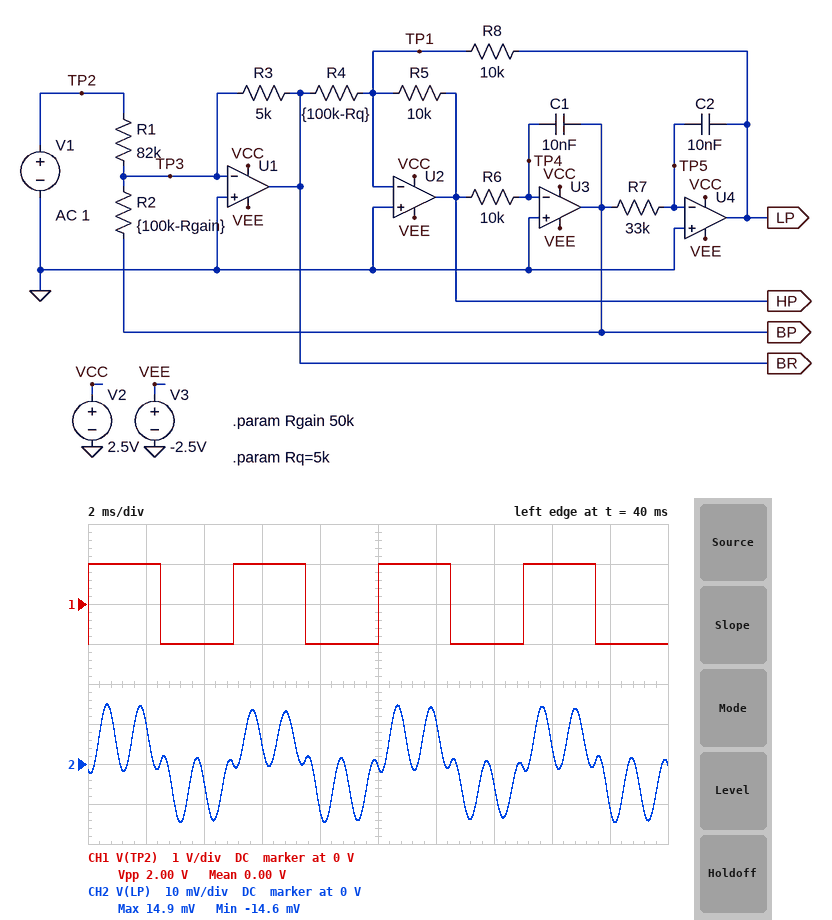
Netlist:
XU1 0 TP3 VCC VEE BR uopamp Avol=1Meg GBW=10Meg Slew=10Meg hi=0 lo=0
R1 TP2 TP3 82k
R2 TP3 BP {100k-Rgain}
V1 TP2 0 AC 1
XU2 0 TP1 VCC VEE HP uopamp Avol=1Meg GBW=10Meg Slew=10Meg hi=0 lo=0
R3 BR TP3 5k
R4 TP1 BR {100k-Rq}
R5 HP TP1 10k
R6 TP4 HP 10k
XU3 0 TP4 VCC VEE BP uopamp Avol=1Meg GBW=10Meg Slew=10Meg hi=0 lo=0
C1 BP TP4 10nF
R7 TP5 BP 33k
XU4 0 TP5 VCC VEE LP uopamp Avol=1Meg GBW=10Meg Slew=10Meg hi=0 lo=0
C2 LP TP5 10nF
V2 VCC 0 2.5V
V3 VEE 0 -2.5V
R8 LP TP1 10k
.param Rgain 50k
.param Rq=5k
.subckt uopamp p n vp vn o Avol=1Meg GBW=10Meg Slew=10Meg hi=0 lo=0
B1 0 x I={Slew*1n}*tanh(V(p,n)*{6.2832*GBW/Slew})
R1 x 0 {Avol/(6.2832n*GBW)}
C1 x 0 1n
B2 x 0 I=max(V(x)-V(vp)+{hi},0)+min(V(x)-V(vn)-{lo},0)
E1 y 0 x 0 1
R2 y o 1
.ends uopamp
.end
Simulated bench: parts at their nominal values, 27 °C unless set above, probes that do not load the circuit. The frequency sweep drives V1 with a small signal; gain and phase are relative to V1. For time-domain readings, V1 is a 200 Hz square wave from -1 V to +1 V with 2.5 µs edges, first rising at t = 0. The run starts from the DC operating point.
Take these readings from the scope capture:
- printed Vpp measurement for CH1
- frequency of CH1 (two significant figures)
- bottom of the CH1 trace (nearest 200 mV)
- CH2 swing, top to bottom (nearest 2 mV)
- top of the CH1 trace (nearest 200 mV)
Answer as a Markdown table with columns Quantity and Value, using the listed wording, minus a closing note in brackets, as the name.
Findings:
| Quantity | Value |
|---|---|
| printed Vpp measurement for CH1 | 2.00 V |
| frequency of CH1 | 200 Hz |
| bottom of the CH1 trace | -1.0 V |
| CH2 swing, top to bottom | 30 mV |
| top of the CH1 trace | 1.0 V |
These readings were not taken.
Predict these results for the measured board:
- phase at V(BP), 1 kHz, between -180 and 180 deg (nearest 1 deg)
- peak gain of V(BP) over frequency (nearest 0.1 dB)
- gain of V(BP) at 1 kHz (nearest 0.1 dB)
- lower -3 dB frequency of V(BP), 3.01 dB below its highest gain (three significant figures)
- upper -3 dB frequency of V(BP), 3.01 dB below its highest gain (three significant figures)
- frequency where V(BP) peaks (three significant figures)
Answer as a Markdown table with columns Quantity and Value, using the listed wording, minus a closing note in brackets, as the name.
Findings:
| Quantity | Value |
|---|---|
| phase at V(BP), 1 kHz, between -180 and 180 deg | 94 deg |
| peak gain of V(BP) over frequency | -4.1 dB |
| gain of V(BP) at 1 kHz | -27.2 dB |
| lower -3 dB frequency of V(BP), 3.01 dB below its highest gain | 868 Hz |
| upper -3 dB frequency of V(BP), 3.01 dB below its highest gain | 884 Hz |
| frequency where V(BP) peaks | 876 Hz |
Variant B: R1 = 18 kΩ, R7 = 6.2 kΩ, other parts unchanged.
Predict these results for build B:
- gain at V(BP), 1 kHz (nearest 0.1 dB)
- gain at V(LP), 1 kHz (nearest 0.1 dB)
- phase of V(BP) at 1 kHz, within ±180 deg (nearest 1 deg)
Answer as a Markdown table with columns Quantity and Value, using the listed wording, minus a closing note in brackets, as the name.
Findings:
| Quantity | Value |
|---|---|
| gain at V(BP), 1 kHz | -36.4 dB |
| gain at V(LP), 1 kHz | -28.2 dB |
| phase of V(BP) at 1 kHz, within ±180 deg | -90 deg |
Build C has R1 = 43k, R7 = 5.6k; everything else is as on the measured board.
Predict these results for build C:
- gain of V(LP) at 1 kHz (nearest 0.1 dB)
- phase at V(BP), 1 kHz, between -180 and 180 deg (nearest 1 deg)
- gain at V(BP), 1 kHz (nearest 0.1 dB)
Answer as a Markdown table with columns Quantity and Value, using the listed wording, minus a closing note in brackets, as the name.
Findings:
| Quantity | Value |
|---|---|
| gain of V(LP) at 1 kHz | -36.1 dB |
| phase at V(BP), 1 kHz, between -180 and 180 deg | -90 deg |
| gain at V(BP), 1 kHz | -45.1 dB |
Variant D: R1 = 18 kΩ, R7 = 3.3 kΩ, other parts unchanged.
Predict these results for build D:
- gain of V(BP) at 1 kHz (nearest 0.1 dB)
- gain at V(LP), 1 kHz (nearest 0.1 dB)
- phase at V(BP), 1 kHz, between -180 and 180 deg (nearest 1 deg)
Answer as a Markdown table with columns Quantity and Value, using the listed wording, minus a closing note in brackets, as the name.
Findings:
| Quantity | Value |
|---|---|
| gain of V(BP) at 1 kHz | -43.1 dB |
| gain at V(LP), 1 kHz | -29.5 dB |
| phase at V(BP), 1 kHz, between -180 and 180 deg | -90 deg |
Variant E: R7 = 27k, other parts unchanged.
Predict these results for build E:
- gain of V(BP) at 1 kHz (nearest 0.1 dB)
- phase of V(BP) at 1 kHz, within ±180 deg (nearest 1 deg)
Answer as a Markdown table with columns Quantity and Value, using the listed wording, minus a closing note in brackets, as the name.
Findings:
| Quantity | Value |
|---|---|
| gain of V(BP) at 1 kHz | -16.0 dB |
| phase of V(BP) at 1 kHz, within ±180 deg | 105 deg |
